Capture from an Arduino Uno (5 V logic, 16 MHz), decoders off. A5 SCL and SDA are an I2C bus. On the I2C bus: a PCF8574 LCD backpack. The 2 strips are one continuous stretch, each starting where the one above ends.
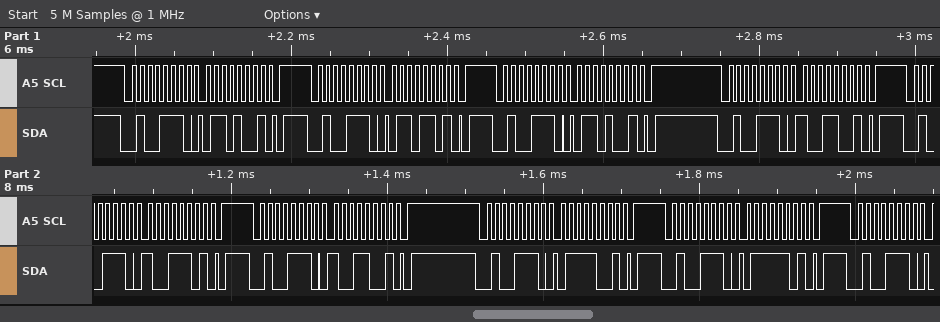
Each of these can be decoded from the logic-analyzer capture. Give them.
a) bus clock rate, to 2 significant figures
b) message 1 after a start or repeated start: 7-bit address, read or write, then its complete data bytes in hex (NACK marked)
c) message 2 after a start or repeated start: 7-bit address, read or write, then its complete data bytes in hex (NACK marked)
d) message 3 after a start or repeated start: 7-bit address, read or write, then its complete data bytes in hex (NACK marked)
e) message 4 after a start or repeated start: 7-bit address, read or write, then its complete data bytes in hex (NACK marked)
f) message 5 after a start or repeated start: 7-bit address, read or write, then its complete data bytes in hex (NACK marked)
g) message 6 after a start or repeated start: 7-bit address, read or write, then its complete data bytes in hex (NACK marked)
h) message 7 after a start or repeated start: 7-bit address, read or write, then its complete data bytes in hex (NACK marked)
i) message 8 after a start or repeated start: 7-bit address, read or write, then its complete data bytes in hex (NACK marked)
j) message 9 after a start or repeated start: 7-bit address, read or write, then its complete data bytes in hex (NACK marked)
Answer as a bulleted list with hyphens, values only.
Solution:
- 100 kHz
- 0x27 write: 69
- 0x27 write: 6D
- 0x27 write: 69
- 0x27 write: 99
- 0x27 write: 9D
- 0x27 write: 99
- 0x27 write: 79
- 0x27 write: 7D
- 0x27 write
